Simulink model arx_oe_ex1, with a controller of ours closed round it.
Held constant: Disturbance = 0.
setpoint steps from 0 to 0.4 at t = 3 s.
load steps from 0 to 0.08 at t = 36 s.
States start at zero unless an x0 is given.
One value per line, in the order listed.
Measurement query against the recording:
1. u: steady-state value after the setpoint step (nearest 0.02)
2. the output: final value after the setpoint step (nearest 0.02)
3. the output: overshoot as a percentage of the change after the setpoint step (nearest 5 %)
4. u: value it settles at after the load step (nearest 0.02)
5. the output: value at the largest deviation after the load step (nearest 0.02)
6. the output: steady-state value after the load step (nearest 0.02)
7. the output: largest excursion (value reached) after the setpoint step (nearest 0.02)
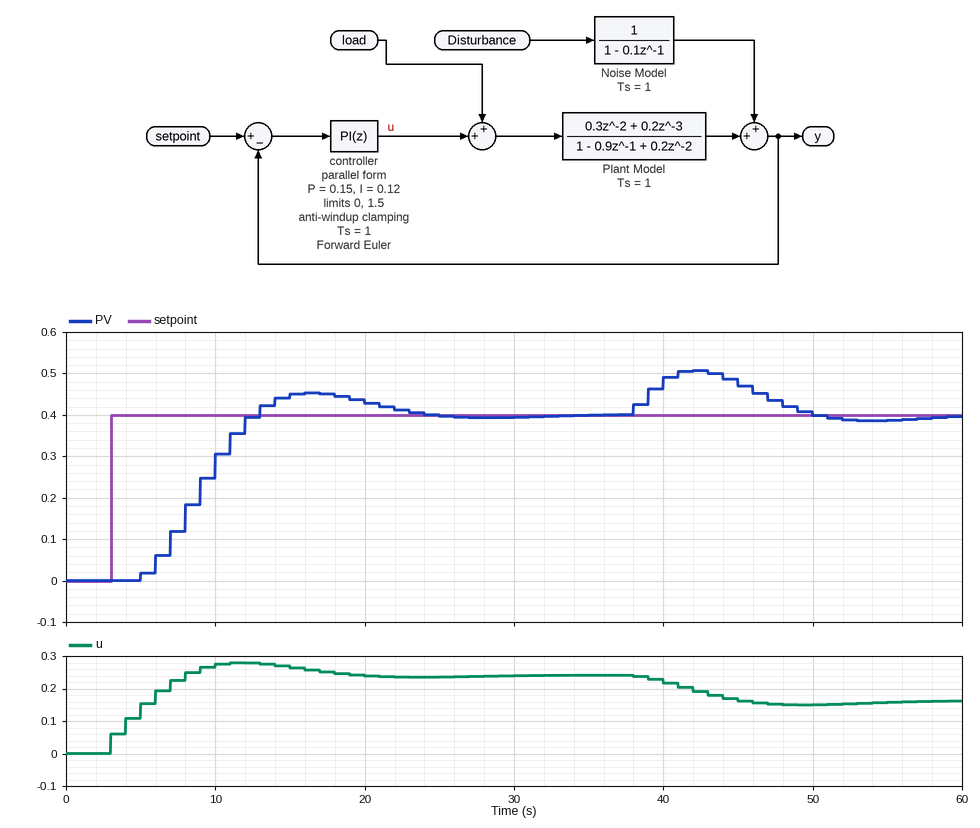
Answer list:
0.24
0.40
15 %
0.16
0.50
0.40
0.46
